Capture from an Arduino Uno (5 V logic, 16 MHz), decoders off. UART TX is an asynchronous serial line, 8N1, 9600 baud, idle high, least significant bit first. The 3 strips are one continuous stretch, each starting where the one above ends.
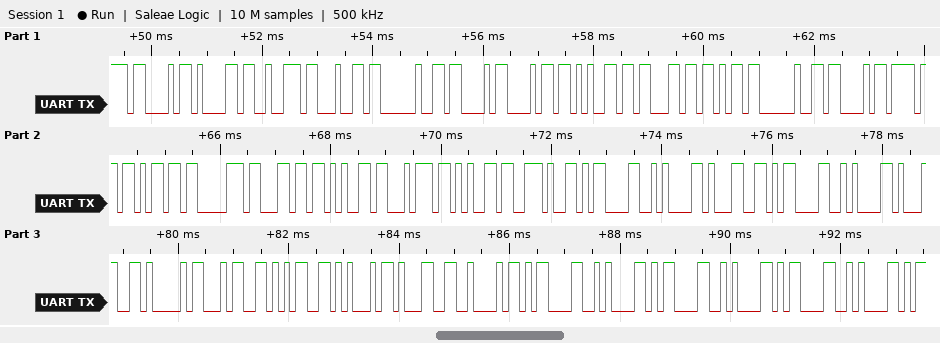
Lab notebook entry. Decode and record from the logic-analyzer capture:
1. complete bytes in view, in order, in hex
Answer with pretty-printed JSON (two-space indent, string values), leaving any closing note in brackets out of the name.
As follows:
{
  "complete bytes in view, in order, in hex": "43 61 72 64 20 43 68 65 63 6B 20 43 6F 6D 70 6C 65 74 65 2E 0D 0A 31 0D 0A 31 41 34 35 45 31 42 0D 0A 0D 0A 0D 0A"
}
